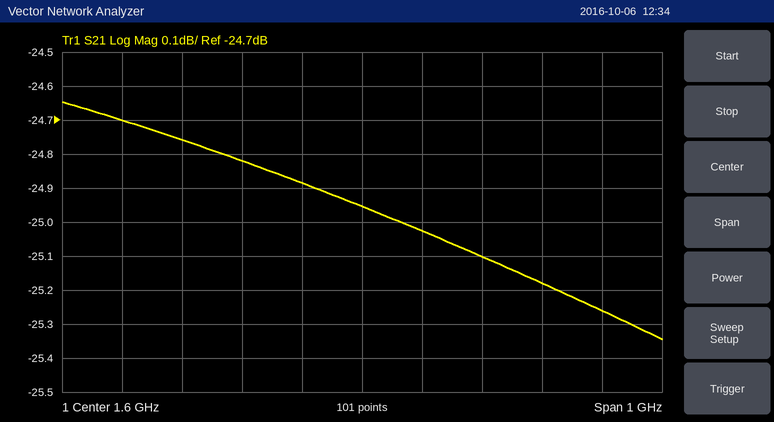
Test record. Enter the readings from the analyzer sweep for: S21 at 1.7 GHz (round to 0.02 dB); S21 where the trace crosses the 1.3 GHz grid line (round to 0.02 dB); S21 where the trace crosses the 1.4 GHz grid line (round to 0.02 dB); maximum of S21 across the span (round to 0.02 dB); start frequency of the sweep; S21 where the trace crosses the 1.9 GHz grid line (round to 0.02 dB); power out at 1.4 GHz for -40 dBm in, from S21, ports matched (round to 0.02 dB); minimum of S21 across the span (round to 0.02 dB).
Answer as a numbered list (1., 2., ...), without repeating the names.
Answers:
1. -25.02 dB
2. -24.76 dB
3. -24.82 dB
4. -24.64 dB
5. 1.1 GHz
6. -25.18 dB
7. -64.82 dBm
8. -25.34 dB
